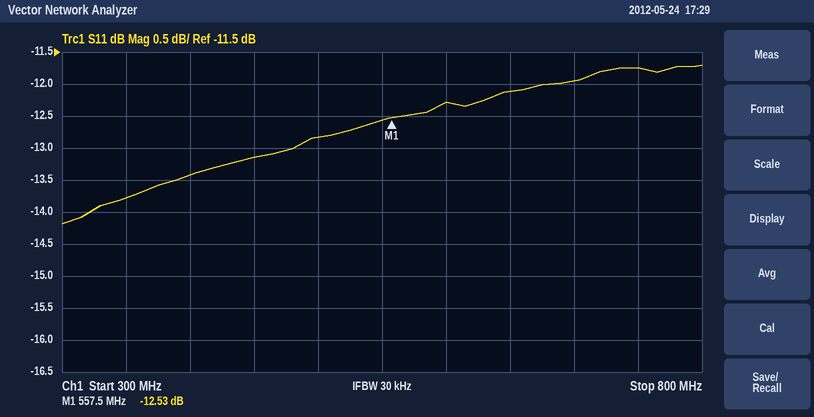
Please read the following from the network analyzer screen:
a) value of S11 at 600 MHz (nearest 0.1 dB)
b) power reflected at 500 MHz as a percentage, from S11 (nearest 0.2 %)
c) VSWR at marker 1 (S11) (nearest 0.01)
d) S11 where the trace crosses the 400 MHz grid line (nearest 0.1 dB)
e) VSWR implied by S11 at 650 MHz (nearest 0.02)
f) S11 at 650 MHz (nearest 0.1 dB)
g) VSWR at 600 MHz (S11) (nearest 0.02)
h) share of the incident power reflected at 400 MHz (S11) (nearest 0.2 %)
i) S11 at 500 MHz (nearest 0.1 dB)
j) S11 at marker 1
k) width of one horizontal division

-12.3 dB
5.2 %
1.62
-13.4 dB
1.66
-12.1 dB
1.64
4.6 %
-12.8 dB
-12.53 dB
50 MHz
